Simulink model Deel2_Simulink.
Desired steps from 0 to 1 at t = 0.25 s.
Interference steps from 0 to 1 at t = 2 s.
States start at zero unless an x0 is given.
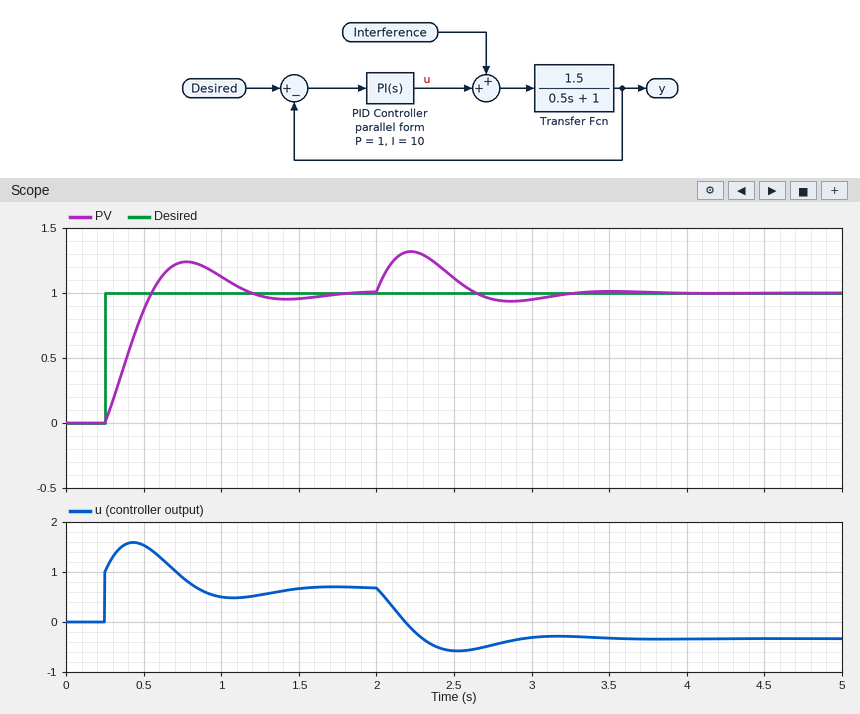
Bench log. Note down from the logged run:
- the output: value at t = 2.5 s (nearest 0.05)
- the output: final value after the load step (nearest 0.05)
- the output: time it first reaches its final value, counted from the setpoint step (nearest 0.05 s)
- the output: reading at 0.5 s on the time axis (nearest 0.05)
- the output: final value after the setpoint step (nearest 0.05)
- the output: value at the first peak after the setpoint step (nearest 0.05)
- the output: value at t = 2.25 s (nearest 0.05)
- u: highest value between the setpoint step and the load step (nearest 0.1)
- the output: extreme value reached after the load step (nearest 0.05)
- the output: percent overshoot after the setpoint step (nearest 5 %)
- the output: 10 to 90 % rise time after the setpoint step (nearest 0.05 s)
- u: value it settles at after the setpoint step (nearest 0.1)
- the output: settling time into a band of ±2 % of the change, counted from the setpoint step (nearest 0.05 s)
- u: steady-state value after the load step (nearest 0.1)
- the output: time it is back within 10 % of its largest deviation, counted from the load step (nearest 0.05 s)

1.10
1.00
0.30 s
0.85
1.00
1.25
1.30
1.6
1.30
25 %
0.25 s
0.7
1.45 s
-0.3
1.10 s
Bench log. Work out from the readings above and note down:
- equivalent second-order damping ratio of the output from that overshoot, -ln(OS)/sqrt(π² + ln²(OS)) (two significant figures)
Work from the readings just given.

0.40
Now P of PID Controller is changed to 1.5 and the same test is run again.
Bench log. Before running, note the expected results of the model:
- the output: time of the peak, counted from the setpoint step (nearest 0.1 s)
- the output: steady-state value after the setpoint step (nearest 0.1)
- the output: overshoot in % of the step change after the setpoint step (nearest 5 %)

0.5 s
1.0
15 %
